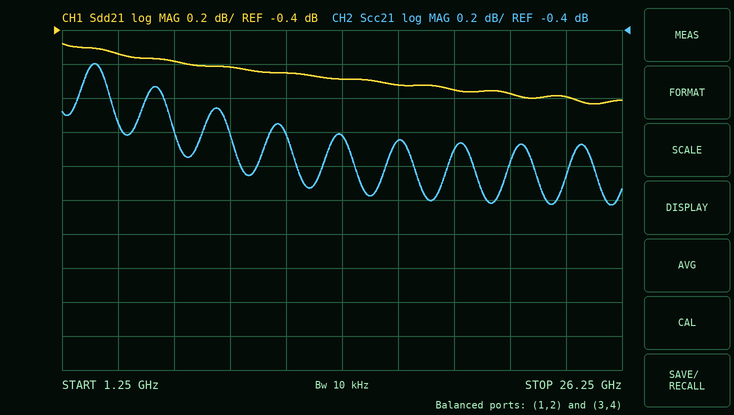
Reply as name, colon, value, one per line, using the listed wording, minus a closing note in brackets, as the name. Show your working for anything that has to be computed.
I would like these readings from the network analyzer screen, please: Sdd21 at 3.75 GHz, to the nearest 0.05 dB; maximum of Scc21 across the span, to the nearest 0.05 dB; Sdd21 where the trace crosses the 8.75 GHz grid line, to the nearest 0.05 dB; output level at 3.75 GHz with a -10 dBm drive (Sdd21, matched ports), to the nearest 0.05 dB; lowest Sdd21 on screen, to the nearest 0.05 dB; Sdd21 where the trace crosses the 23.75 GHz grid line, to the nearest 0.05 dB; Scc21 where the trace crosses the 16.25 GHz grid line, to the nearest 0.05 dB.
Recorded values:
Sdd21 at 3.75 GHz, to the nearest 0.05 dB: -0.55 dB
maximum of Scc21 across the span, to the nearest 0.05 dB: -0.60 dB
Sdd21 where the trace crosses the 8.75 GHz grid line, to the nearest 0.05 dB: -0.60 dB
output level at 3.75 GHz with a -10 dBm drive (Sdd21, matched ports), to the nearest 0.05 dB: -10 dBm + (-0.55 dB) = -10.55 dBm
lowest Sdd21 on screen, to the nearest 0.05 dB: -0.85 dB
Sdd21 where the trace crosses the 23.75 GHz grid line, to the nearest 0.05 dB: -0.80 dB
Scc21 where the trace crosses the 16.25 GHz grid line, to the nearest 0.05 dB: -1.05 dB
